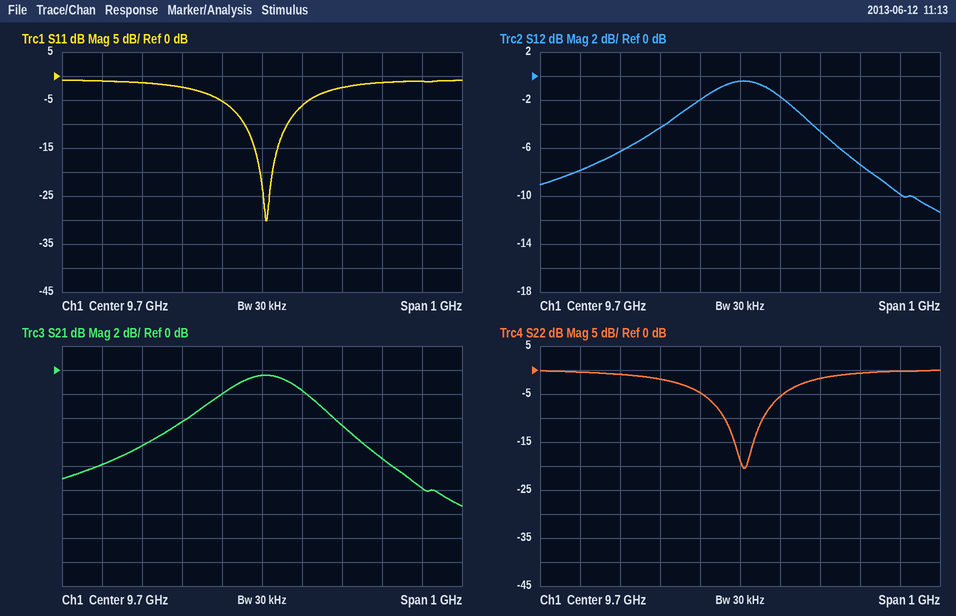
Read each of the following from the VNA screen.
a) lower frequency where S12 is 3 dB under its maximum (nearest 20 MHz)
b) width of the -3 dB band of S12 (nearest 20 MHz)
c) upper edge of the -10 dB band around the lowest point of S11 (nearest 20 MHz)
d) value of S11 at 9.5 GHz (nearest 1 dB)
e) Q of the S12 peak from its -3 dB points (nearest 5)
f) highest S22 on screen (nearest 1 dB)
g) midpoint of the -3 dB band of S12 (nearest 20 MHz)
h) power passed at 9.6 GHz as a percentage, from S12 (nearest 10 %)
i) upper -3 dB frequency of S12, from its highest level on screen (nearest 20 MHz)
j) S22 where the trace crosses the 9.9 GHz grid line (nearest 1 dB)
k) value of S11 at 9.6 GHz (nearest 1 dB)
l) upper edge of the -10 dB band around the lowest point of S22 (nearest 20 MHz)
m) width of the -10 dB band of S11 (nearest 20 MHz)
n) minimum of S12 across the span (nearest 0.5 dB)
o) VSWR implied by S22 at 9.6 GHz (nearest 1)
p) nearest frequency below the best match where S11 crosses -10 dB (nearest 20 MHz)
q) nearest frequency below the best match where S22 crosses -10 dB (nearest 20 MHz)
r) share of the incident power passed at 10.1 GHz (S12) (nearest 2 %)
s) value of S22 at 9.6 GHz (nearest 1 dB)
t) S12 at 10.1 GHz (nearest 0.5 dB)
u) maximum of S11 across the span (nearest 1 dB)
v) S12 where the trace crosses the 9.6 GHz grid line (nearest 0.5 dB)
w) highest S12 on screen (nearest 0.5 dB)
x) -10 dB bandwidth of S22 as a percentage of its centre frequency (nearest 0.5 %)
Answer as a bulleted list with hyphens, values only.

- 9.54 GHz
- 320 MHz
- 9.76 GHz
- -2 dB
- 30
- 0 dB
- 9.70 GHz
- 60 %
- 9.86 GHz
- -2 dB
- -5 dB
- 9.76 GHz
- 100 MHz
- -11.5 dB
- 4
- 9.66 GHz
- 9.66 GHz
- 10 %
- -5 dB
- -10.0 dB
- -1 dB
- -2.0 dB
- -0.5 dB
- 1.0 %
